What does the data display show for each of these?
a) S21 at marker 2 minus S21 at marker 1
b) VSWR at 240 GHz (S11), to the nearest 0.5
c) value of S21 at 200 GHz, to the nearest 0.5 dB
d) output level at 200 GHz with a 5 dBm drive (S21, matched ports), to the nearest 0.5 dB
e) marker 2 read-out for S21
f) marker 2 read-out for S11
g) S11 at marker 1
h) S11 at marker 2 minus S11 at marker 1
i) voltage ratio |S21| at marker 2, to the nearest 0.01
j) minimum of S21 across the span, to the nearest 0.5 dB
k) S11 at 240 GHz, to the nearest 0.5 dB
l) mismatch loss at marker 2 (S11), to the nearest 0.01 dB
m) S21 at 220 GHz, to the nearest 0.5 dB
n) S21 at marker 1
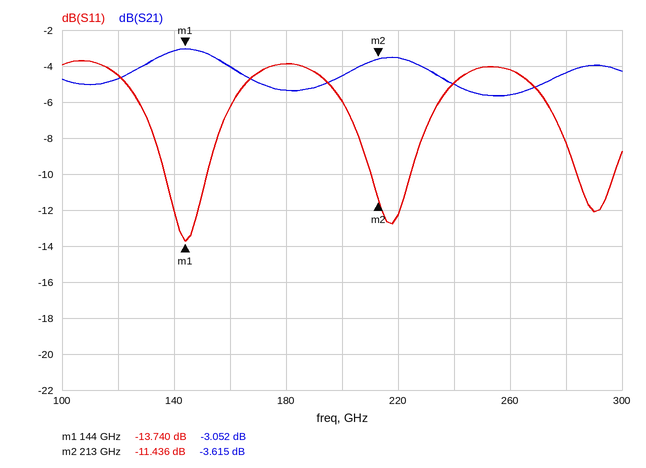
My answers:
-0.563 dB
3.5
-4.5 dB
0.5 dBm
-3.615 dB
-11.436 dB
-13.740 dB
2.304 dB
0.66
-5.5 dB
-5.0 dB
0.32 dB
-3.5 dB
-3.052 dB
